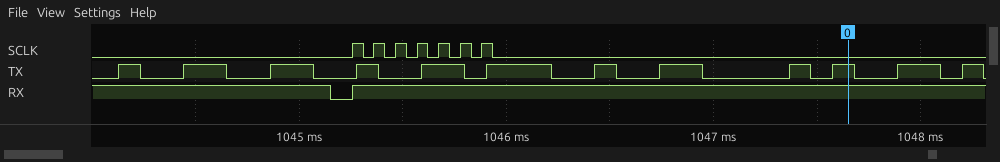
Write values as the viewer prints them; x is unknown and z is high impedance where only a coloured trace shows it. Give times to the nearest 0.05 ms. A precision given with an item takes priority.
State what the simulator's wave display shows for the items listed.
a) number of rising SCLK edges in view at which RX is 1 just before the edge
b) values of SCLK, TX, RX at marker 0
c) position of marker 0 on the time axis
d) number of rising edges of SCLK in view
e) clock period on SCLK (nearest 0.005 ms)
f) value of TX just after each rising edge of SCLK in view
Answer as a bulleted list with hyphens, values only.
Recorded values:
- 6
- SCLK=0, TX=1, RX=1
- 1047.65 ms
- 7
- 0.105 ms
- 0 1 0 0 1 1 0
